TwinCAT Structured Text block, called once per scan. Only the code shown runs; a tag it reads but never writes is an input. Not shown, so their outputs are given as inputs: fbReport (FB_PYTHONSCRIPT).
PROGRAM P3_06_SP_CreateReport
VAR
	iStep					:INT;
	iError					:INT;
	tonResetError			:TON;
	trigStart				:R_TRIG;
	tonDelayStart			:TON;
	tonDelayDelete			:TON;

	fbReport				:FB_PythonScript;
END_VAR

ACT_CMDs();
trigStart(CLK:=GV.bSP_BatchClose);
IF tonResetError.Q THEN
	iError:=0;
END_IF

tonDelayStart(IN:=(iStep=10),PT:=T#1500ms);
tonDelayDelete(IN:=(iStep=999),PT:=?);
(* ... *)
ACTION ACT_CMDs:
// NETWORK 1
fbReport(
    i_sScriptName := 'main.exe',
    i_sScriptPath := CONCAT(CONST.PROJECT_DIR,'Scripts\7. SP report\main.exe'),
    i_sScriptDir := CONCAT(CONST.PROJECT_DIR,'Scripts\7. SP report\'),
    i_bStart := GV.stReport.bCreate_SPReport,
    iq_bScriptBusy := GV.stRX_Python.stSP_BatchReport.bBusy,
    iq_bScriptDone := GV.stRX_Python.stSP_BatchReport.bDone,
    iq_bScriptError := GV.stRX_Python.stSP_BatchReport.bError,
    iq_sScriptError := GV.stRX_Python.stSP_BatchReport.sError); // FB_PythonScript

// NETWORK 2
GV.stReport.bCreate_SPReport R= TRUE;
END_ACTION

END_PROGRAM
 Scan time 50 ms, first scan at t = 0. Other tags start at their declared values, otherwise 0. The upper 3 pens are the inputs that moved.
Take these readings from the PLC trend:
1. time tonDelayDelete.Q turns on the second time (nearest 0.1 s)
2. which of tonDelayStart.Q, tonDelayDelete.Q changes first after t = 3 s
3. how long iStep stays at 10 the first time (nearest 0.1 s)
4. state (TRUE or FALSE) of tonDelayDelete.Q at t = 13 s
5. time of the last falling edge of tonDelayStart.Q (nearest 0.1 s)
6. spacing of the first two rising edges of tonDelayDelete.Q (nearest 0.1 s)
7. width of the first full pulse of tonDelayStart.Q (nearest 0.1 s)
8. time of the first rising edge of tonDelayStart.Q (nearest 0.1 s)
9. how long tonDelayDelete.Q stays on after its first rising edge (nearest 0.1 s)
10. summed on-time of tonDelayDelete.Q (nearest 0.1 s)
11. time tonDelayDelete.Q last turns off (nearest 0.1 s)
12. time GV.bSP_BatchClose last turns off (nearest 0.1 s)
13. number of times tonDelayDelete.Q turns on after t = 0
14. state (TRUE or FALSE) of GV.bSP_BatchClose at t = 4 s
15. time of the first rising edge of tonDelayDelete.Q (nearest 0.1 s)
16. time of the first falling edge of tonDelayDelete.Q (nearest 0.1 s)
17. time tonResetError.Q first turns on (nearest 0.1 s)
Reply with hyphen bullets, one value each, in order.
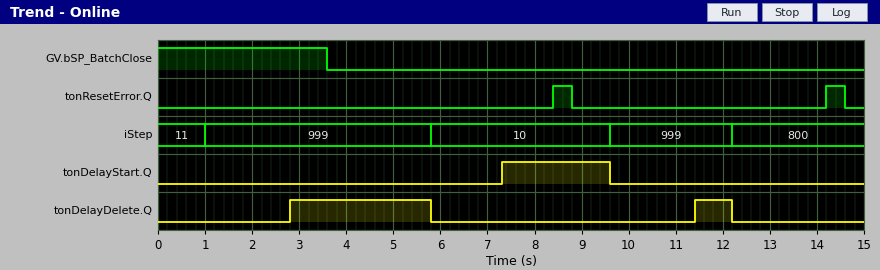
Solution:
- 11.4 s
- tonDelayDelete.Q
- 3.8 s
- FALSE
- 9.6 s
- 8.6 s
- 2.3 s
- 7.3 s
- 3.0 s
- 3.8 s
- 12.2 s
- 3.6 s
- 2
- FALSE
- 2.8 s
- 5.8 s
- 8.4 s
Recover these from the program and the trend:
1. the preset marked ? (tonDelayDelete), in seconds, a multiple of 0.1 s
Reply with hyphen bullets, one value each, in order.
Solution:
- 1.8 s
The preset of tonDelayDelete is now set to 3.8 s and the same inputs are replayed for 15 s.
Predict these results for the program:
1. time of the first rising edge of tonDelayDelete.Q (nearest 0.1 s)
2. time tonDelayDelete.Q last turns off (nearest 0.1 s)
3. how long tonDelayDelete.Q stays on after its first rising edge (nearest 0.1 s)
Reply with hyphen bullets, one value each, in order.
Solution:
- 4.8 s
- 5.8 s
- 1.0 s
